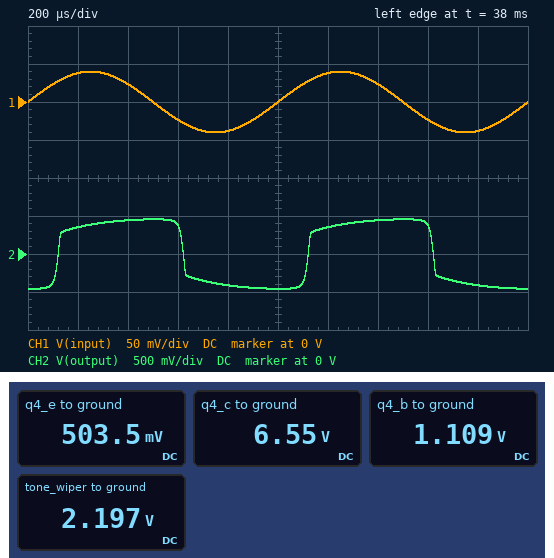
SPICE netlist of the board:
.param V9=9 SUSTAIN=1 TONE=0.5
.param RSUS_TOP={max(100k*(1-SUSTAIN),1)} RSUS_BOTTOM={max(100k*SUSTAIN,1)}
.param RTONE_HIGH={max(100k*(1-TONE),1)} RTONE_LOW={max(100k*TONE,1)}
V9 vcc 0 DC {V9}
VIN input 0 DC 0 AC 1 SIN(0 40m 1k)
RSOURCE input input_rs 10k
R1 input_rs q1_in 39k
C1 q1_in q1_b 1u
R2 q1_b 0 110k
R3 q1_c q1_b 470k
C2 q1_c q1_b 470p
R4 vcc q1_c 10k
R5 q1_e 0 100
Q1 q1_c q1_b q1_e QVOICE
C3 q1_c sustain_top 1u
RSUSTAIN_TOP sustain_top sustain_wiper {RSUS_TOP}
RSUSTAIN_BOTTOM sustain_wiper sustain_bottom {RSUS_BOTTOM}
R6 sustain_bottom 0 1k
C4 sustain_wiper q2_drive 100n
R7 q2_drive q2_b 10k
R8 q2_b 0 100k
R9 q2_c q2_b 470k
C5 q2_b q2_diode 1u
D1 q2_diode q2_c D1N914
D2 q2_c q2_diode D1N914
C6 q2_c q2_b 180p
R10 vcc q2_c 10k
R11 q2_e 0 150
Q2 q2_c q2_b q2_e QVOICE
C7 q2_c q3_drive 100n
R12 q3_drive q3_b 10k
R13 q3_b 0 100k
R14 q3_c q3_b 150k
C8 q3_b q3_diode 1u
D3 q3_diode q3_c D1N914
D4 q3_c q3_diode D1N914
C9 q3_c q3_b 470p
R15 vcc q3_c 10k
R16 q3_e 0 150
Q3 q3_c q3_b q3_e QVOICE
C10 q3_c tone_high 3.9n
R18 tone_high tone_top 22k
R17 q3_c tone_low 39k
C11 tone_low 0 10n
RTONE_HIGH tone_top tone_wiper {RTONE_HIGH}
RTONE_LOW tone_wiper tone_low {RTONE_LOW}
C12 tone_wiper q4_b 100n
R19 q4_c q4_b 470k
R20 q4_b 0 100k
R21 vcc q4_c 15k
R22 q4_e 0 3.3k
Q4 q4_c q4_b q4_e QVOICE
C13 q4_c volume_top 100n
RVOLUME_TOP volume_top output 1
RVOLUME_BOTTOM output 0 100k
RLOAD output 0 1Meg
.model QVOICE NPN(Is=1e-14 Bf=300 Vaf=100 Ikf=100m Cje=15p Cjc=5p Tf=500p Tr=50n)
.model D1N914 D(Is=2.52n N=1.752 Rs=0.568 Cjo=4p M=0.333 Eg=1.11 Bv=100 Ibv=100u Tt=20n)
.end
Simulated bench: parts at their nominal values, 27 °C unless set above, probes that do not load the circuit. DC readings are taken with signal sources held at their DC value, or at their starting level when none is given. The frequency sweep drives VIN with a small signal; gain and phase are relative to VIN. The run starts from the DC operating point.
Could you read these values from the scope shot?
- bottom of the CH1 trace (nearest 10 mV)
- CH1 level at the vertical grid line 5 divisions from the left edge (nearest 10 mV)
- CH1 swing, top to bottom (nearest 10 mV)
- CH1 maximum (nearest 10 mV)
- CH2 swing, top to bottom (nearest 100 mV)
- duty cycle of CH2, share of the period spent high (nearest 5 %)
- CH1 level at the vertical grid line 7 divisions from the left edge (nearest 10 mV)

-40 mV
0 V
80 mV
40 mV
900 mV
50 %
20 mV
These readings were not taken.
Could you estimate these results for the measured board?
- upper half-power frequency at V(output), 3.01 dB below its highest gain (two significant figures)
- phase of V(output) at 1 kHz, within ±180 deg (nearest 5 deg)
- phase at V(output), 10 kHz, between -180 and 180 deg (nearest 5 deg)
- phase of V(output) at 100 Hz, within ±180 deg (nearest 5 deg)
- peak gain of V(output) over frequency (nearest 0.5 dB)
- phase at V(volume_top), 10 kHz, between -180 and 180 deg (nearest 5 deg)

850 Hz
-70 deg
145 deg
90 deg
59.0 dB
145 deg
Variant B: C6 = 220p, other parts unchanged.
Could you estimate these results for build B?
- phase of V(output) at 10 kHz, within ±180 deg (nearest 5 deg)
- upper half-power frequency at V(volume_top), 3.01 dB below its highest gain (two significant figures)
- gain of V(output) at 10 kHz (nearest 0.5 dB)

140 deg
840 Hz
20.0 dB
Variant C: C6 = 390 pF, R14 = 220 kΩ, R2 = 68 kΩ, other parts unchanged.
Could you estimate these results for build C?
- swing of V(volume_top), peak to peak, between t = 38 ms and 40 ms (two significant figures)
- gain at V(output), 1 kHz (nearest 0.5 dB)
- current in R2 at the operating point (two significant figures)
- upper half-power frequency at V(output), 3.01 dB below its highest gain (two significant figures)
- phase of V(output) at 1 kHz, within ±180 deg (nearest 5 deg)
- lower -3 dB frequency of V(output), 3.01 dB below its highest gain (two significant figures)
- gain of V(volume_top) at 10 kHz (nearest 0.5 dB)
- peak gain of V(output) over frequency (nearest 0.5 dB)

910 mV
55.5 dB
9.7 µA
780 Hz
-85 deg
98 Hz
16.0 dB
60.5 dB
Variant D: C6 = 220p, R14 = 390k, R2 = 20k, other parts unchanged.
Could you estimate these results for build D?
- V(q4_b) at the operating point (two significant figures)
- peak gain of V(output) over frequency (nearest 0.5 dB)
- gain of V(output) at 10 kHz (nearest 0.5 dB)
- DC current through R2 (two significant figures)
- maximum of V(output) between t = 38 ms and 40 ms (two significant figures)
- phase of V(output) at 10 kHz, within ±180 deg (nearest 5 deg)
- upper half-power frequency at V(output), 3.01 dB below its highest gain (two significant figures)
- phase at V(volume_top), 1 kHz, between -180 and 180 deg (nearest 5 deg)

1.1 V
2.5 dB
-5.0 dB
18 µA
47 mV
85 deg
5.8 kHz
-170 deg
